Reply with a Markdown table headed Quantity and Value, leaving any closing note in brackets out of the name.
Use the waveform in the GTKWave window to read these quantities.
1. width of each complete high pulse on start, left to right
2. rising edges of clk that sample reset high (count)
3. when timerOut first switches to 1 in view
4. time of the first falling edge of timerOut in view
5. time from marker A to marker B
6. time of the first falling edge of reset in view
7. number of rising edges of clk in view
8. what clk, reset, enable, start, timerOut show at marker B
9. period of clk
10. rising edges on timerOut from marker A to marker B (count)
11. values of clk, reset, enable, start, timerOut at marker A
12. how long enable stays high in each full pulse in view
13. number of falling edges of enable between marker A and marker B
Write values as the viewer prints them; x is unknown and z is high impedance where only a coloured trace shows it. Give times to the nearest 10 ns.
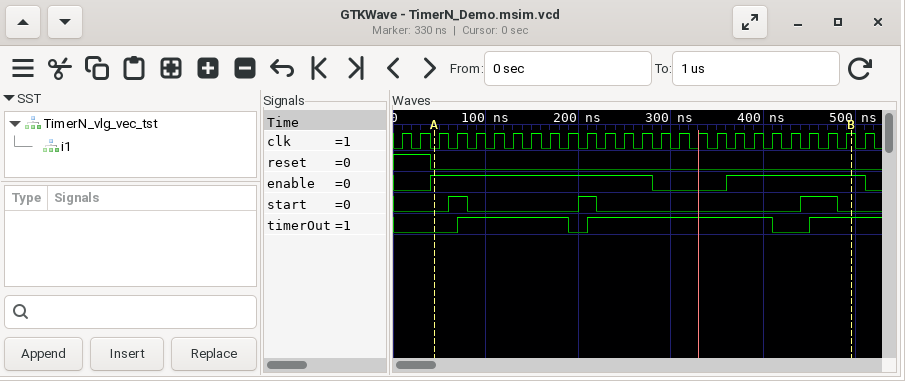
| Quantity | Value |
|---|---|
| width of each complete high pulse on start, left to right | 20 ns, 20 ns, 40 ns |
| rising edges of clk that sample reset high | 2 |
| when timerOut first switches to 1 in view | 70 ns |
| time of the first falling edge of timerOut in view | 190 ns |
| time from marker A to marker B | 450 ns |
| time of the first falling edge of reset in view | 40 ns |
| number of rising edges of clk in view | 26 |
| what clk, reset, enable, start, timerOut show at marker B | clk=1, reset=0, enable=1, start=0, timerOut=1 |
| period of clk | 20 ns |
| rising edges on timerOut from marker A to marker B | 3 |
| values of clk, reset, enable, start, timerOut at marker A | clk=0, reset=0, enable=1, start=0, timerOut=0 |
| how long enable stays high in each full pulse in view | 240 ns, 150 ns |
| number of falling edges of enable between marker A and marker B | 1 |
